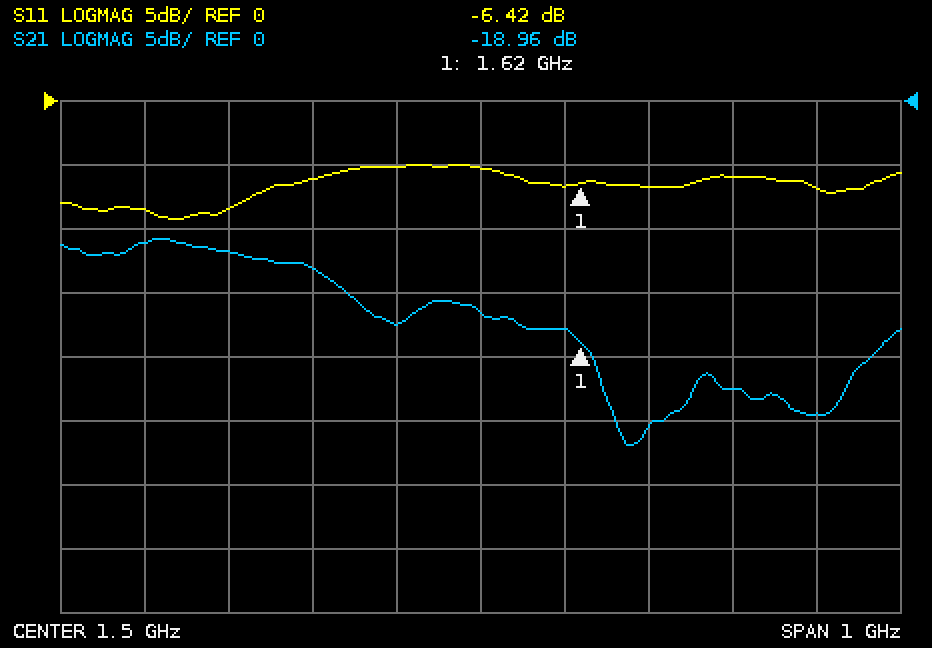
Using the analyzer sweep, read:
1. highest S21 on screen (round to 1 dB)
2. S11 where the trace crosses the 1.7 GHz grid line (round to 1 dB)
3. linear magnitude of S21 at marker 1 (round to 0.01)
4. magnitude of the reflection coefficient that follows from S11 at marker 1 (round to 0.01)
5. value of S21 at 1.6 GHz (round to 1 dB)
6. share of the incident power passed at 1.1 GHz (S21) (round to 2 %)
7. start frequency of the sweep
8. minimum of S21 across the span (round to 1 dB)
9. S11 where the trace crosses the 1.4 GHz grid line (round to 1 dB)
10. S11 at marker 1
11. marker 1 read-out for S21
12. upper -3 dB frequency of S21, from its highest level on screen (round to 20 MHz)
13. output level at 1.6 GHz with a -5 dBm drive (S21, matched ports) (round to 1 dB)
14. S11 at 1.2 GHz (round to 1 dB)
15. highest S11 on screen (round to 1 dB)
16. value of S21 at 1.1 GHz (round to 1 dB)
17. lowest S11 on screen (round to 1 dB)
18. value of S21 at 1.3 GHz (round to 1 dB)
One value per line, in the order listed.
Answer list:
-11 dB
-7 dB
0.11
0.48
-18 dB
8 %
1 GHz
-27 dB
-5 dB
-6.42 dB
-18.96 dB
1.32 GHz
-23 dBm
-8 dB
-5 dB
-11 dB
-9 dB
-13 dB
